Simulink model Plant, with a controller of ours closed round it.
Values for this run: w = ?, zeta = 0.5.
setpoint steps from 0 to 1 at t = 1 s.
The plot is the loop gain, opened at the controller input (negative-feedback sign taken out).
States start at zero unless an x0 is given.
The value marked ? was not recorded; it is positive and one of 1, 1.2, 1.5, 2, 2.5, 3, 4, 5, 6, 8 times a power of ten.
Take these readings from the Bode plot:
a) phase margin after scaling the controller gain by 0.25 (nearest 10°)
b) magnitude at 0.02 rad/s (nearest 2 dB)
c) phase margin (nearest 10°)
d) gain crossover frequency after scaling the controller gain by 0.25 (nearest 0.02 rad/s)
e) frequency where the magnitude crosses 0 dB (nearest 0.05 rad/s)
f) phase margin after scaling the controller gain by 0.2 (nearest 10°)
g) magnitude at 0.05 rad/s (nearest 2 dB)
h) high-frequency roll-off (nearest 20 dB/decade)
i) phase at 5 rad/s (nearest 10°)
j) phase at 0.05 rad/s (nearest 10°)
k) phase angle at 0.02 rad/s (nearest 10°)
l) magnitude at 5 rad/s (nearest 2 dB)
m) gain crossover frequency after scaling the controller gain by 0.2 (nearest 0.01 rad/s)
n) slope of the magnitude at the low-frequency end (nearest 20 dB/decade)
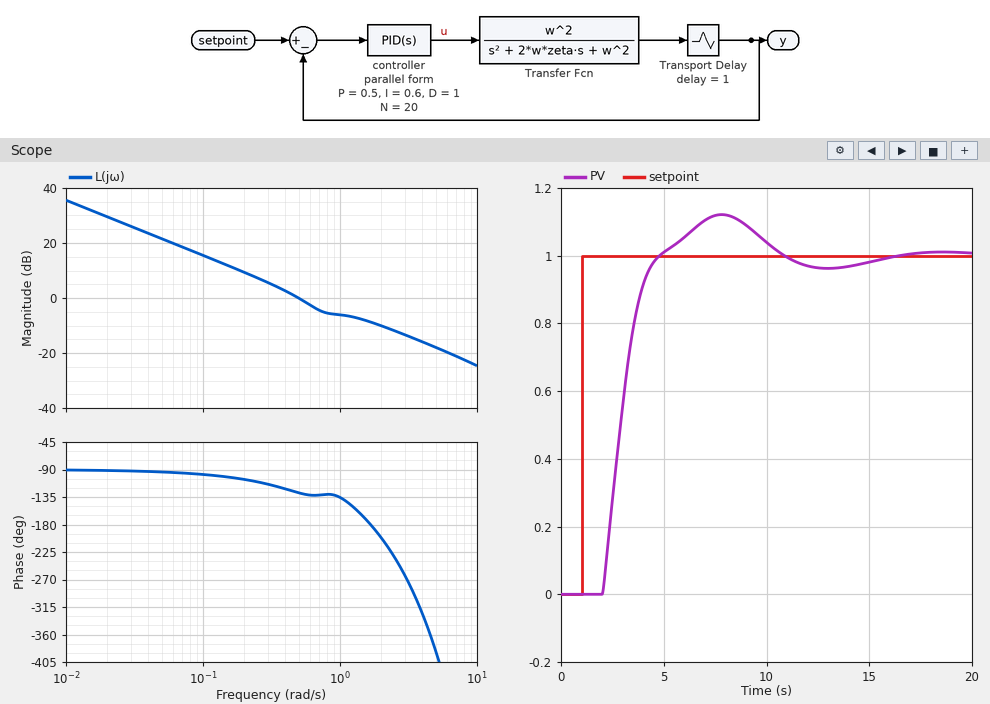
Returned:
80°
30 dB
50°
0.14 rad/s
0.50 rad/s
80°
22 dB
-20 dB/decade
-390°
-90°
-90°
-18 dB
0.12 rad/s
-20 dB/decade
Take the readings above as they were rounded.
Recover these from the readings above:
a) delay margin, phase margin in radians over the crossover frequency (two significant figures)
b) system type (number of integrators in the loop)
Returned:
1.7 s
1
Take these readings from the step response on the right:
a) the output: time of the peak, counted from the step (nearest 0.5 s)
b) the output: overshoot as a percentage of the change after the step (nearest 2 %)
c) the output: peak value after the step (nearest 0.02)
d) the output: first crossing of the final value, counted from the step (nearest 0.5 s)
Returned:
7.0 s
12 %
1.12
4.0 s
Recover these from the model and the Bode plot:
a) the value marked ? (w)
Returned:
0.8
